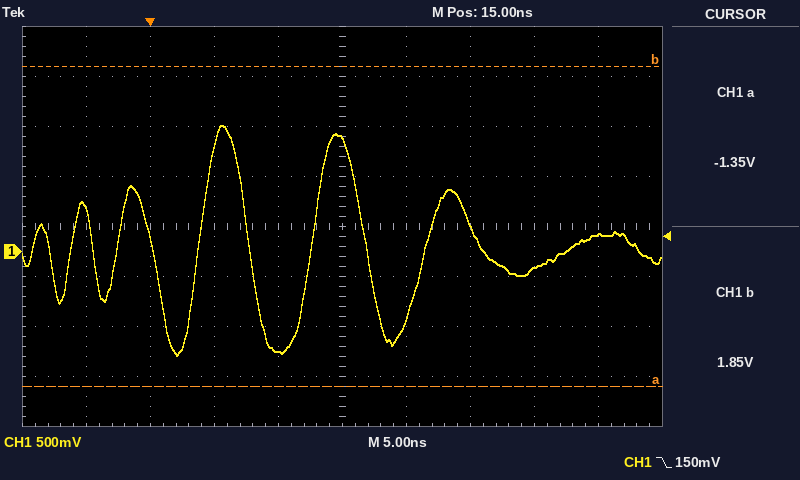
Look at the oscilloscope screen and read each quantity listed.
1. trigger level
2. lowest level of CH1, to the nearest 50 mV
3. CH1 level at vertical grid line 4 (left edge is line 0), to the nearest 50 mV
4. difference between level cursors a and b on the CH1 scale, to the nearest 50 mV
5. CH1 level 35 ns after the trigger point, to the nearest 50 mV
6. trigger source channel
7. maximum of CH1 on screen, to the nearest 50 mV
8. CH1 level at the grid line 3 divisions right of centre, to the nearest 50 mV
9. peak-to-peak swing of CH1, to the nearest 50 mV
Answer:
150 mV
-1.05 V
-1.00 V
3.20 V
150 mV
CH1
1.25 V
-150 mV
2.30 V
